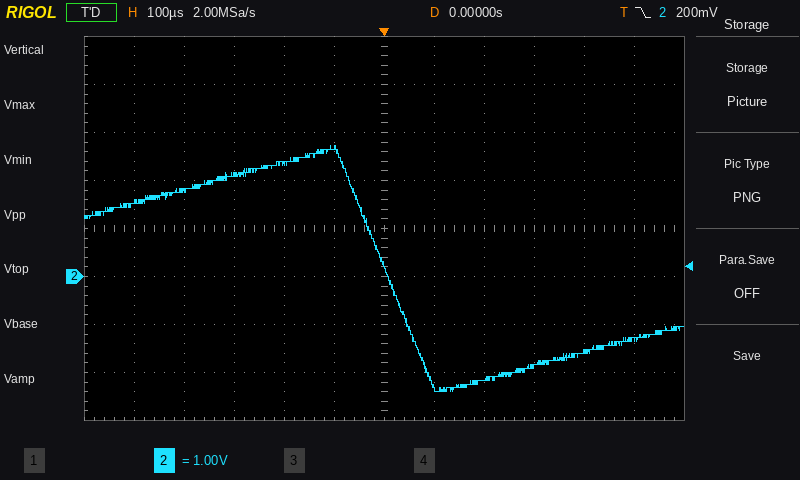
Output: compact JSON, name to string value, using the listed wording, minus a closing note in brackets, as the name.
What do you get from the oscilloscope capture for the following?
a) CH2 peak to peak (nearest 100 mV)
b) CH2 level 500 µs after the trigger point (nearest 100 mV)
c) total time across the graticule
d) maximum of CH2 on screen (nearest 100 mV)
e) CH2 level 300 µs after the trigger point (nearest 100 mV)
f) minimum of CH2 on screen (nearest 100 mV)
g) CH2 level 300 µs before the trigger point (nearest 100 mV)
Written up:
{"CH2 peak to peak": "5.1 V", "CH2 level 500 µs after the trigger point": "-1.3 V", "total time across the graticule": "1.2 ms", "maximum of CH2 on screen": "2.7 V", "CH2 level 300 µs after the trigger point": "-1.9 V", "minimum of CH2 on screen": "-2.4 V", "CH2 level 300 µs before the trigger point": "2.1 V"}
